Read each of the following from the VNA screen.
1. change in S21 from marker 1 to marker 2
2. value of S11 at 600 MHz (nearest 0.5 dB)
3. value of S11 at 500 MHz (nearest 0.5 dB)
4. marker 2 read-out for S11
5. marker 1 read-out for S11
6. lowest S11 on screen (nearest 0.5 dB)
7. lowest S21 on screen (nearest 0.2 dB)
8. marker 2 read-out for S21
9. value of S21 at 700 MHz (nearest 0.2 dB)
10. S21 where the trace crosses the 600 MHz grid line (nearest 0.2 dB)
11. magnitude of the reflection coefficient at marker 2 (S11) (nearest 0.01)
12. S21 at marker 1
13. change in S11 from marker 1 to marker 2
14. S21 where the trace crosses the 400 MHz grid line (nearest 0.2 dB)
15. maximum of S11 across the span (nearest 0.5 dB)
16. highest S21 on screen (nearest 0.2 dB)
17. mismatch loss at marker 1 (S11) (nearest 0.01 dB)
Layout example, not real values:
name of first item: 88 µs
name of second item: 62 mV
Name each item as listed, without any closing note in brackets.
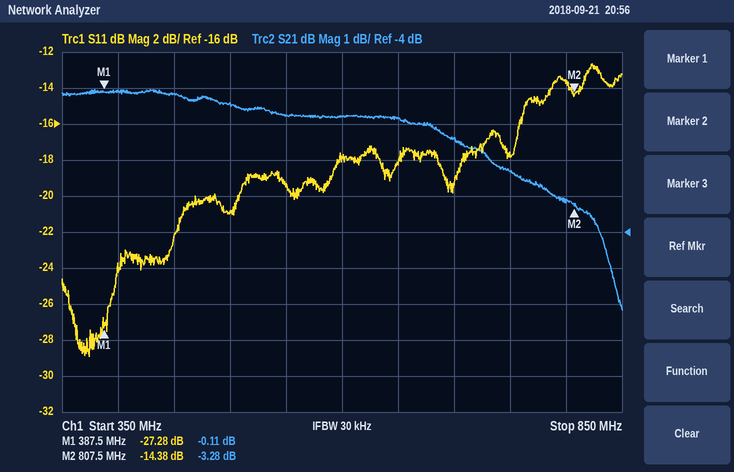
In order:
change in S21 from marker 1 to marker 2: -3.17 dB
value of S11 at 600 MHz: -18.0 dB
value of S11 at 500 MHz: -21.0 dB
marker 2 read-out for S11: -14.38 dB
marker 1 read-out for S11: -27.28 dB
lowest S11 on screen: -29.0 dB
lowest S21 on screen: -6.2 dB
marker 2 read-out for S21: -3.28 dB
value of S21 at 700 MHz: -1.4 dB
S21 where the trace crosses the 600 MHz grid line: -0.8 dB
magnitude of the reflection coefficient at marker 2 (S11): 0.19
S21 at marker 1: -0.11 dB
change in S11 from marker 1 to marker 2: 12.90 dB
S21 where the trace crosses the 400 MHz grid line: 0.0 dB
maximum of S11 across the span: -12.5 dB
highest S21 on screen: 0.0 dB
mismatch loss at marker 1 (S11): 0.01 dB
